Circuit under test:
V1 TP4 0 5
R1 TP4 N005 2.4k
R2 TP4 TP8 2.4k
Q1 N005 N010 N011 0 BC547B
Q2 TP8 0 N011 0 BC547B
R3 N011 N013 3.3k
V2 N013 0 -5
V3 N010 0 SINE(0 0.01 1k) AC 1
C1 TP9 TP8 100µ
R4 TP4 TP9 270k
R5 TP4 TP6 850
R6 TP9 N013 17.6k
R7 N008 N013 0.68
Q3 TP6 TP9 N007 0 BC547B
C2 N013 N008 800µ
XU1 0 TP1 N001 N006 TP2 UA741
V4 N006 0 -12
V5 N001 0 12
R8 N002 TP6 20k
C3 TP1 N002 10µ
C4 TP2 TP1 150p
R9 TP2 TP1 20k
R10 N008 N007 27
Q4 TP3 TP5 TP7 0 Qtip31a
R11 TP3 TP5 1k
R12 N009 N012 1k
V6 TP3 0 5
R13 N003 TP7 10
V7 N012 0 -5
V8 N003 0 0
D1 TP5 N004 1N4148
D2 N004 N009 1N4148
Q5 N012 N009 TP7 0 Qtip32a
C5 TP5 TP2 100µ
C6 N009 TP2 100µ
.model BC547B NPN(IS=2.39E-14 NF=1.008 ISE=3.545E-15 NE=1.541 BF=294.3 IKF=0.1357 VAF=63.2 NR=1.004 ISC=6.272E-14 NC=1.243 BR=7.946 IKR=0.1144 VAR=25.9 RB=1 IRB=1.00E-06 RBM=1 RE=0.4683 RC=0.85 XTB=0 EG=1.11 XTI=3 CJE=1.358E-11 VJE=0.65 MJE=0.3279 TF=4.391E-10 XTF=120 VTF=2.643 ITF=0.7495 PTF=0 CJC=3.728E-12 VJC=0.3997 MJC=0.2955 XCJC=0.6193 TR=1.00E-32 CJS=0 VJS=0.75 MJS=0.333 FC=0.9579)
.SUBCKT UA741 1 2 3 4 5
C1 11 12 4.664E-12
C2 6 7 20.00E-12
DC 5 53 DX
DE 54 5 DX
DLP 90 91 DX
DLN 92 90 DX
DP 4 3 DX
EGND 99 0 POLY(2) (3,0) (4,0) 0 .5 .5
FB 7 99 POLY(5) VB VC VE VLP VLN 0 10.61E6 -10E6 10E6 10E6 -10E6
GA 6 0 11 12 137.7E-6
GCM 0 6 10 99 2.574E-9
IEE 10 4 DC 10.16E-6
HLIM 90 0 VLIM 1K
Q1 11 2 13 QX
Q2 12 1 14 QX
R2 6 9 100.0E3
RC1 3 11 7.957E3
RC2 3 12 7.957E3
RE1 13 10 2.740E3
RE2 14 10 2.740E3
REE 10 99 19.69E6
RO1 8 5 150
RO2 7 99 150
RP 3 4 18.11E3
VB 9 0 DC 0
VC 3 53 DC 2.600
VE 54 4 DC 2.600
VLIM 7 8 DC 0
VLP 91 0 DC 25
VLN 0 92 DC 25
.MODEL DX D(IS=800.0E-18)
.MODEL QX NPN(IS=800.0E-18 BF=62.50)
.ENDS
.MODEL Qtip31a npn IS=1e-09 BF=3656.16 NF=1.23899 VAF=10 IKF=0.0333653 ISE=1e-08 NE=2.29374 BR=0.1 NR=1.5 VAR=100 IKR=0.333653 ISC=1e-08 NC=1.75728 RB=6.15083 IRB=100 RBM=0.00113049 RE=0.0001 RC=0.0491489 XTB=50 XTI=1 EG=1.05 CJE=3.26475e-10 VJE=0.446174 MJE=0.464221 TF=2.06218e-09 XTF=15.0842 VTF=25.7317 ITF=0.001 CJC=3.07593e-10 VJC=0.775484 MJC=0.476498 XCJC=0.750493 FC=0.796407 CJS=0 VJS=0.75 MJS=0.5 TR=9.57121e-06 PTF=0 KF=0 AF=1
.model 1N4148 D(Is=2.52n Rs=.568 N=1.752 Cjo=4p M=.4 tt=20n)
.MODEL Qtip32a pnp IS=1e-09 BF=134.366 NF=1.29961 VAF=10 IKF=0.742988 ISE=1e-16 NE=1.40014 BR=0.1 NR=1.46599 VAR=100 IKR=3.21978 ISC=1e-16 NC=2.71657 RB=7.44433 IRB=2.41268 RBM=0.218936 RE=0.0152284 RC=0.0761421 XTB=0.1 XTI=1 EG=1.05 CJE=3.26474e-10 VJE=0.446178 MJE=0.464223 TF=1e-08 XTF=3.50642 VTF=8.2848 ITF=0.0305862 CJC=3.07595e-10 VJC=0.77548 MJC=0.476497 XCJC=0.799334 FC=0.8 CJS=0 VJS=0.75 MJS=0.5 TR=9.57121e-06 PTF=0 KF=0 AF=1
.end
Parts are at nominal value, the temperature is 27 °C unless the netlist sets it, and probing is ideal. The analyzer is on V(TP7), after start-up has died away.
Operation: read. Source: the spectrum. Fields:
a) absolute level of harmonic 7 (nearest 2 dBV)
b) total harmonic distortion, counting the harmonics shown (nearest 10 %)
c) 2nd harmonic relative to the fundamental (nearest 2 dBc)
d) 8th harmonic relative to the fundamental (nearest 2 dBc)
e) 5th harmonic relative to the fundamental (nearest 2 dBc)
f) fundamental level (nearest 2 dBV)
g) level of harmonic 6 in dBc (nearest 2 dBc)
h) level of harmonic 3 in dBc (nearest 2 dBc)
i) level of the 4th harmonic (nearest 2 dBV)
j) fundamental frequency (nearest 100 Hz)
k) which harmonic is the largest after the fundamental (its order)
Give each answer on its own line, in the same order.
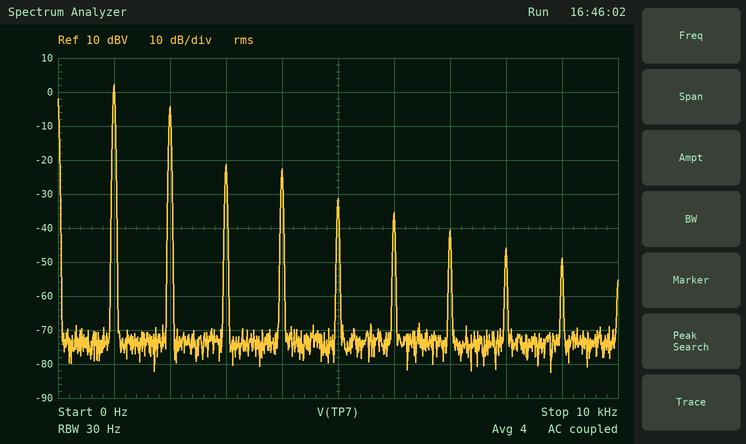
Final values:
-40 dBV
50 %
-6 dBc
-48 dBc
-34 dBc
2 dBV
-38 dBc
-24 dBc
-22 dBV
1.0 kHz
2
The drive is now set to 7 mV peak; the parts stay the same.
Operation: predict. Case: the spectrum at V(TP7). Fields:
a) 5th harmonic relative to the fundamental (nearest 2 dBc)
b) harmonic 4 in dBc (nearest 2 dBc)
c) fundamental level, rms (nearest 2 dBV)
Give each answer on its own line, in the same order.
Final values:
-36 dBc
-28 dBc
-2 dBV
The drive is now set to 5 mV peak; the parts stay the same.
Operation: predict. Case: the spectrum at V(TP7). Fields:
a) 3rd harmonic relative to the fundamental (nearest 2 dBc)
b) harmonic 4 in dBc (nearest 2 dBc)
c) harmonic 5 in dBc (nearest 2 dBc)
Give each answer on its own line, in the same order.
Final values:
-26 dBc
-30 dBc
-42 dBc
